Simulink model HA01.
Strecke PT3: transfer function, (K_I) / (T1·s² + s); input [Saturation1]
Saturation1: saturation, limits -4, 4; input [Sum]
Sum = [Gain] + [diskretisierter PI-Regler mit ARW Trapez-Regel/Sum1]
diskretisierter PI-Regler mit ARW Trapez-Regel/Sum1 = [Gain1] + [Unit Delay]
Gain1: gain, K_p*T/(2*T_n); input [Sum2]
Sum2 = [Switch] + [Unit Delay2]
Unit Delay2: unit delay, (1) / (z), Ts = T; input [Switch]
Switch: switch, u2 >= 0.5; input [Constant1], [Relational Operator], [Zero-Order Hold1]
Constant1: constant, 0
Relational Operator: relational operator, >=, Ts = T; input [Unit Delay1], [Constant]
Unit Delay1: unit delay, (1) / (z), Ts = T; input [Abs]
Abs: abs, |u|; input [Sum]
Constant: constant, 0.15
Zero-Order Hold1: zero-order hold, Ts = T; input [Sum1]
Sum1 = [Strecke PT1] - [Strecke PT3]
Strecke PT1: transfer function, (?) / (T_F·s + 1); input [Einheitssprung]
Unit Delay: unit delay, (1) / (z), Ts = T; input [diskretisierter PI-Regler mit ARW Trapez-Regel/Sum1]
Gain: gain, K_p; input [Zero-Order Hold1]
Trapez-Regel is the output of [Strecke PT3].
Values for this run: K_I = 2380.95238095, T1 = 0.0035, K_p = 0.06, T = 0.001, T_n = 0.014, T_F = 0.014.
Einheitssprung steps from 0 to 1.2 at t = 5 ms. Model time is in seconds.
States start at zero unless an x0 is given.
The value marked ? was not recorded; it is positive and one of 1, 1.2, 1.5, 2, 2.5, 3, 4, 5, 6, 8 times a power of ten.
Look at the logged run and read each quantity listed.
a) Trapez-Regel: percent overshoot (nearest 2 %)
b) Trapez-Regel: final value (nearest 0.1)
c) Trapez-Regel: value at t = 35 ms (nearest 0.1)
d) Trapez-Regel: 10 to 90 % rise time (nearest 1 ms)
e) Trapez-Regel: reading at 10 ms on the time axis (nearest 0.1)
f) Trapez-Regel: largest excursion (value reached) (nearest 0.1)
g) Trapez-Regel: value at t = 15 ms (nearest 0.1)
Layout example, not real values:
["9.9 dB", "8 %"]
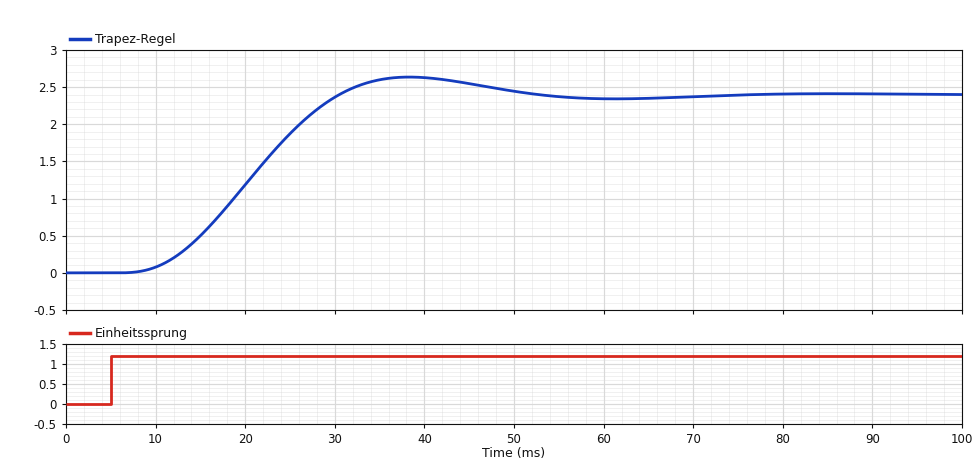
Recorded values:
["10 %", "2.4", "2.6", "15 ms", "0.1", "2.6", "0.5"]
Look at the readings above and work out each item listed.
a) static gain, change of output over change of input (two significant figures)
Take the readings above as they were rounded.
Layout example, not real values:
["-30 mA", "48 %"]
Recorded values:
["2.0"]
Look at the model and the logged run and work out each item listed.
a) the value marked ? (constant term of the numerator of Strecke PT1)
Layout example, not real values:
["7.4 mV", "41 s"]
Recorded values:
["2"]
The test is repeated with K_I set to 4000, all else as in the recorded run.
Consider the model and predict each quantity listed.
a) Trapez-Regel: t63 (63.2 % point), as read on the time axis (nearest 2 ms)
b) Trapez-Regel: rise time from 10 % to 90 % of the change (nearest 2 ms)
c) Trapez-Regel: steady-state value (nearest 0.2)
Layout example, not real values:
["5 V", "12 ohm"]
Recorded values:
["20 ms", "14 ms", "2.4"]
